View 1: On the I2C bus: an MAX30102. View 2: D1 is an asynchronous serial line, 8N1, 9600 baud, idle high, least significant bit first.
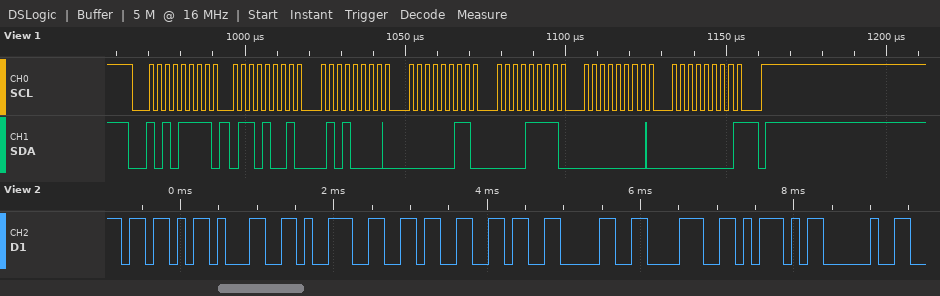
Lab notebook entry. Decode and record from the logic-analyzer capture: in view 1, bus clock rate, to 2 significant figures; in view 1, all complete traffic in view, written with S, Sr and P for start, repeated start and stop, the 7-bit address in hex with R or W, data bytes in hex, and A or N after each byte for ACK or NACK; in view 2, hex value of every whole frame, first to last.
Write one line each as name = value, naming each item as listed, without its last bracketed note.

in view 1, bus clock rate, to 2 significant figures = 400 kHz
in view 1, all complete traffic in view, written with S, Sr and P for start, repeated start and stop, the 7-bit address in hex with R or W, data bytes in hex, and A or N after each byte for ACK or NACK = S 57R A 69 A 50 A 03 A 0F A 00 A 00 N P
in view 2, hex value of every whole frame, first to last = 5B 31 39 36 36 30 38 5D 20
